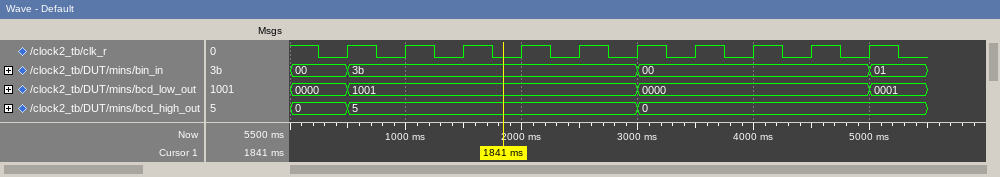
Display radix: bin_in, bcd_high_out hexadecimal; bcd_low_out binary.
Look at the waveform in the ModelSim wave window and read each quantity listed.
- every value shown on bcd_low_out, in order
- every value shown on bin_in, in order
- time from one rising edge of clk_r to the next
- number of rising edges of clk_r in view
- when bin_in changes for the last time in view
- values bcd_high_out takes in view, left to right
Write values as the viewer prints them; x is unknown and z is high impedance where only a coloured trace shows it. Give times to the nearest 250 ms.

0000, 1001, 0000, 0001
00, 3b, 00, 01
500 ms
10
5000 ms
0, 5, 0
